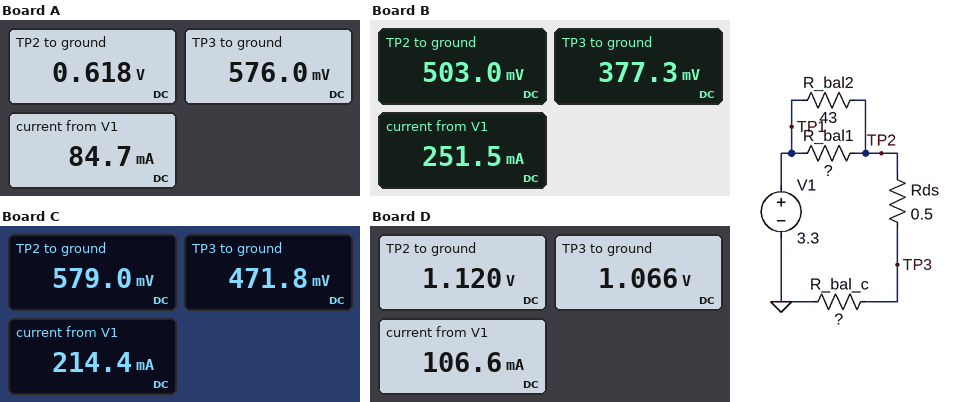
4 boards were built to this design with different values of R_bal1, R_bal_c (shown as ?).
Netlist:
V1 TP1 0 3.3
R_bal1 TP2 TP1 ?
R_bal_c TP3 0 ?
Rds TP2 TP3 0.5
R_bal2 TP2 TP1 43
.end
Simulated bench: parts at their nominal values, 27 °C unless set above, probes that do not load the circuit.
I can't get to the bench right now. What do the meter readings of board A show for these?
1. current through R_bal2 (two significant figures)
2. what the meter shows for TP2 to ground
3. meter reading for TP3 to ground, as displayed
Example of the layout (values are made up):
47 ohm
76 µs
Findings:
62 mA
0.618 V
576.0 mV
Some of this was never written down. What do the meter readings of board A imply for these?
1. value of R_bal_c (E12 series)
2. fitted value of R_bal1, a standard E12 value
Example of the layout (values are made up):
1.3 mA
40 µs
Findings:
6.8 Ω
120 Ω
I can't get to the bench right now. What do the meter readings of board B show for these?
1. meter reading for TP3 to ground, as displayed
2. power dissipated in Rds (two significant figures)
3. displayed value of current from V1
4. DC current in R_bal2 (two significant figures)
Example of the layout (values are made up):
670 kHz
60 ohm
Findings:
377.3 mV
32 mW
251.5 mA
65 mA
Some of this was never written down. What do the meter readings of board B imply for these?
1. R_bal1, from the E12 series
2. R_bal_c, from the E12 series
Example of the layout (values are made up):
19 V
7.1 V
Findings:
15 Ω
1.5 Ω
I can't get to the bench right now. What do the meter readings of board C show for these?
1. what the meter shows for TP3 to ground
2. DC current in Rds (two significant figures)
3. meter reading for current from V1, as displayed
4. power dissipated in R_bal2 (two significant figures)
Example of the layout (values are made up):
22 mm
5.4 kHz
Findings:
471.8 mV
210 mA
214.4 mA
170 mW
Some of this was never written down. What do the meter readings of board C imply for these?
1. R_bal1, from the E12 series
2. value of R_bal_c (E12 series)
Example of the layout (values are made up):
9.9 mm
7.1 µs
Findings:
18 Ω
2.2 Ω
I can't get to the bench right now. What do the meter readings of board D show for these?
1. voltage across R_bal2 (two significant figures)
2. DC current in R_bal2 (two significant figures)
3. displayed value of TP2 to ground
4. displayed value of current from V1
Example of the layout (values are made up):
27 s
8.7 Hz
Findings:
2.2 V
51 mA
1.120 V
106.6 mA
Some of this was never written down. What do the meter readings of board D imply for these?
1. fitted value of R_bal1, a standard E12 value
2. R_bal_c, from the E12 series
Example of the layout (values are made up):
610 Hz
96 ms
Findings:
39 Ω
10 Ω
